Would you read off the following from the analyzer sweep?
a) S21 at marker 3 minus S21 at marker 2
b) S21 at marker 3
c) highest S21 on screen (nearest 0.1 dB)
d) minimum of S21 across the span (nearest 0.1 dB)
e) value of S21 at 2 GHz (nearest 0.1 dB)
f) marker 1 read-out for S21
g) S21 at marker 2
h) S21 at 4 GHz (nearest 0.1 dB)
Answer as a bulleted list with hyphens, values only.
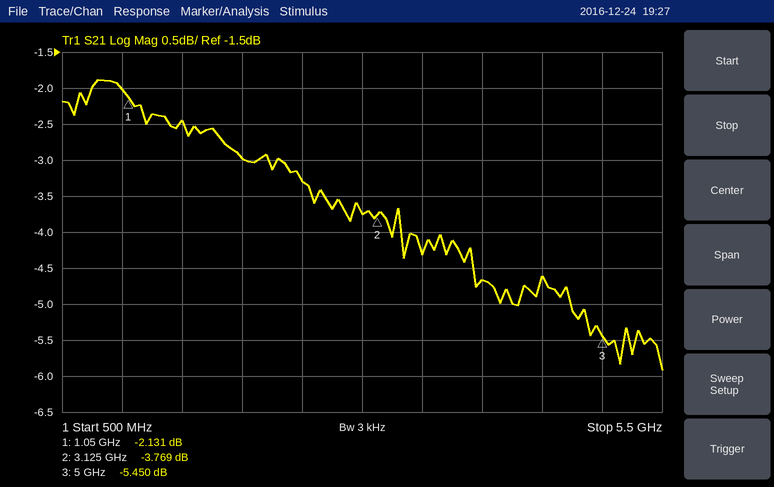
- -1.681 dB
- -5.450 dB
- -1.9 dB
- -5.9 dB
- -3.0 dB
- -2.131 dB
- -3.769 dB
- -4.7 dB
